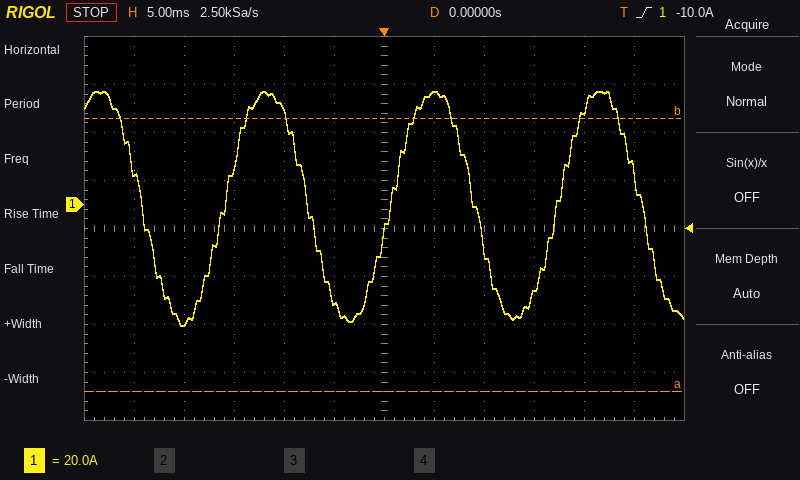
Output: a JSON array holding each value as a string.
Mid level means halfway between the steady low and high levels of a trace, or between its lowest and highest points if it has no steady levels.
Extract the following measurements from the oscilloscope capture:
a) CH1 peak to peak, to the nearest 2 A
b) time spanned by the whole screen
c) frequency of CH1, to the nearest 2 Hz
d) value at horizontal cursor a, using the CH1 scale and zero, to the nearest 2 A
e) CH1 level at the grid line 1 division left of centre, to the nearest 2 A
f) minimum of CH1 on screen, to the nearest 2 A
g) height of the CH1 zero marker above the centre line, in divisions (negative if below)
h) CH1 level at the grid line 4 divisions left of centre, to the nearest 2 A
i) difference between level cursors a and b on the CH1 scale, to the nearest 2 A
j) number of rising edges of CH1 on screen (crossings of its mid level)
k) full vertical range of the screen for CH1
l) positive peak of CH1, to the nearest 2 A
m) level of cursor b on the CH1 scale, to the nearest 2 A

["98 A", "60 ms", "60 Hz", "-78 A", "-40 A", "-50 A", "+0.5 div", "-50 A", "114 A", "3", "160 A", "48 A", "36 A"]
